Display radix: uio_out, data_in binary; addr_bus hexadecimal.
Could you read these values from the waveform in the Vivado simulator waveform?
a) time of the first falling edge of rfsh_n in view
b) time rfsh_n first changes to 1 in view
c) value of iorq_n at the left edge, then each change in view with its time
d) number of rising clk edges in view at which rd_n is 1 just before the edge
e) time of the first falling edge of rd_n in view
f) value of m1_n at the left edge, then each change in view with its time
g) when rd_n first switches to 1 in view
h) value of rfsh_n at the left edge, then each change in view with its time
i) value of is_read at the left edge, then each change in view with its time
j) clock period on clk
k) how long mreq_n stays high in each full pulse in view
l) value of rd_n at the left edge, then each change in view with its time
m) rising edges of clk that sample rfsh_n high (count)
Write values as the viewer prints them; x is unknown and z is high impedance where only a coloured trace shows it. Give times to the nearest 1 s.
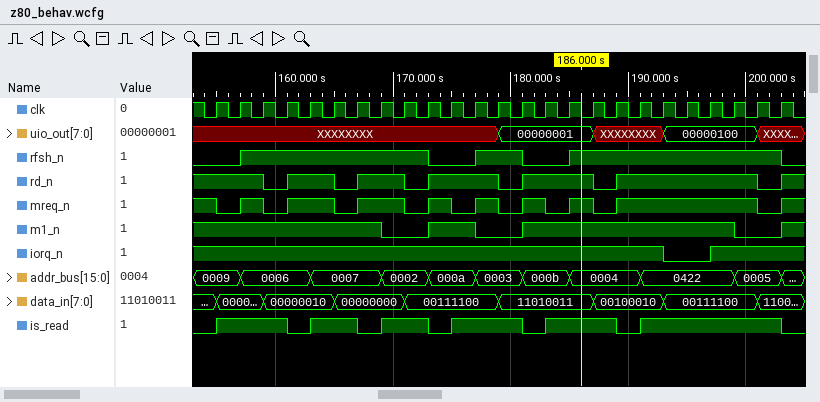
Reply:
173 s
157 s
1, 0 at 193 s, 1 at 197 s
19
159 s
1, 0 at 169 s, 1 at 173 s, 0 at 177 s, 1 at 181 s, 0 at 199 s, 1 at 203 s
161 s
0, 1 at 157 s, 0 at 173 s, 1 at 177 s, 0 at 181 s, 1 at 185 s, 0 at 203 s
0, 1 at 155 s, 0 at 161 s, 1 at 163 s, 0 at 167 s, 1 at 169 s, 0 at 173 s, 1 at 175 s, 0 at 181 s, 1 at 183 s, 0 at 189 s, 1 at 191 s, 0 at 203 s
2 s
2 s, 4 s, 4 s, 2 s, 2 s, 2 s, 2 s, 12 s
1, 0 at 159 s, 1 at 161 s, 0 at 165 s, 1 at 167 s, 0 at 171 s, 1 at 173 s, 0 at 179 s, 1 at 181 s, 0 at 187 s, 1 at 189 s, 0 at 201 s, 1 at 203 s
19
